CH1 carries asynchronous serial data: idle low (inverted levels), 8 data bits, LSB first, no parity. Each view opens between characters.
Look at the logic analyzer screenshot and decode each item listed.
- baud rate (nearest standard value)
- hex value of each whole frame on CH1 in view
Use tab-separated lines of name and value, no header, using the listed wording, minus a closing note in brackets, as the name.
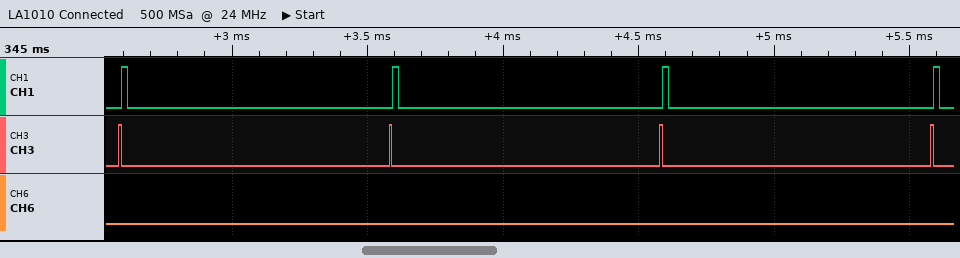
baud rate	38400 baud
hex value of each whole frame on CH1 in view	FF, FF, FF
